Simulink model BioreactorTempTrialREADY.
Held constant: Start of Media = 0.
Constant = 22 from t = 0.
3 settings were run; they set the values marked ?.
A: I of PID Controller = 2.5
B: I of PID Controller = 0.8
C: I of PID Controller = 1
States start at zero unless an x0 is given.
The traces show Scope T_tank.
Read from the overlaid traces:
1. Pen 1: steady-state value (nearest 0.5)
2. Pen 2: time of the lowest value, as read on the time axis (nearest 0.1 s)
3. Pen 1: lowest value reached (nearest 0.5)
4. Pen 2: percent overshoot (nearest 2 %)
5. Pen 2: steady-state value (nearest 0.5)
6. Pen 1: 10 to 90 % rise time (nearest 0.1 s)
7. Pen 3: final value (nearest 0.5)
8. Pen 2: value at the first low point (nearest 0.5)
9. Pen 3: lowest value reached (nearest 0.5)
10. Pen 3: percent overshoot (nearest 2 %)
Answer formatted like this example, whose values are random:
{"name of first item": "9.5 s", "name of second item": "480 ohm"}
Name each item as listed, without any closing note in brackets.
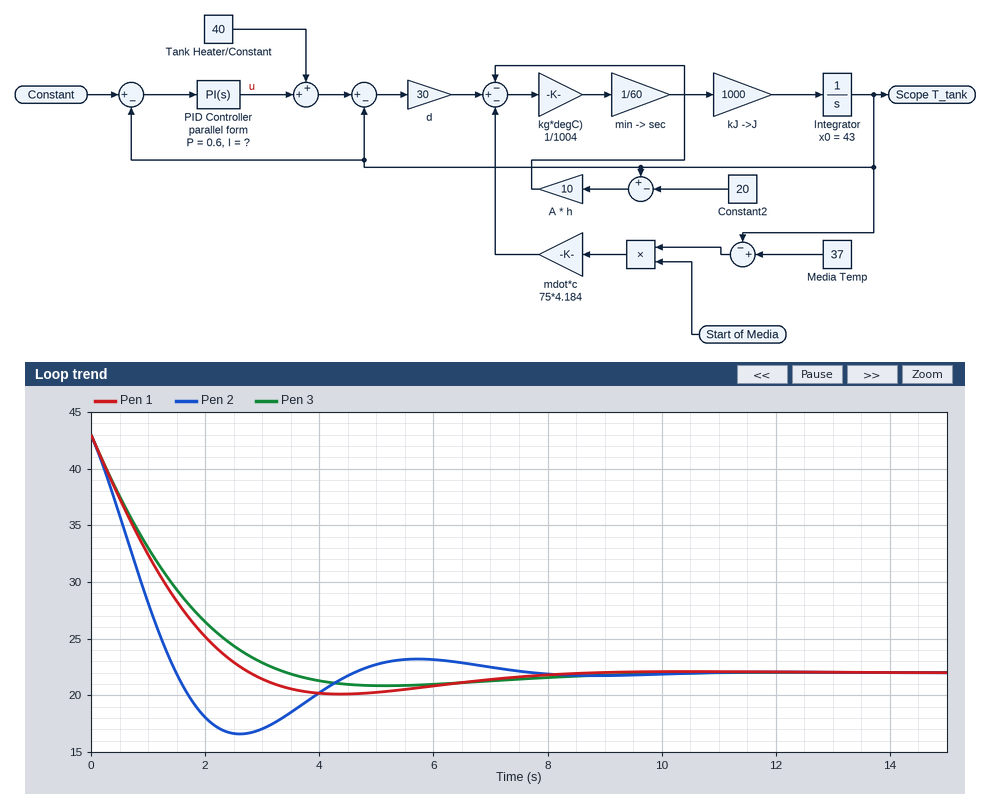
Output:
{"Pen 1: steady-state value": "22.0", "Pen 2: time of the lowest value, as read on the time axis": "2.6 s", "Pen 1: lowest value reached": "20.0", "Pen 2: percent overshoot": "26 %", "Pen 2: steady-state value": "22.0", "Pen 1: 10 to 90 % rise time": "2.0 s", "Pen 3: final value": "22.0", "Pen 2: value at the first low point": "16.5", "Pen 3: lowest value reached": "21.0", "Pen 3: percent overshoot": "6 %"}
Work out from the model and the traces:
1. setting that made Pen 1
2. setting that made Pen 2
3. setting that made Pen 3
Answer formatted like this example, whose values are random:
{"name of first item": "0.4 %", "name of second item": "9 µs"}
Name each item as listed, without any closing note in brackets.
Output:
{"setting that made Pen 1": "C", "setting that made Pen 2": "A", "setting that made Pen 3": "B"}
